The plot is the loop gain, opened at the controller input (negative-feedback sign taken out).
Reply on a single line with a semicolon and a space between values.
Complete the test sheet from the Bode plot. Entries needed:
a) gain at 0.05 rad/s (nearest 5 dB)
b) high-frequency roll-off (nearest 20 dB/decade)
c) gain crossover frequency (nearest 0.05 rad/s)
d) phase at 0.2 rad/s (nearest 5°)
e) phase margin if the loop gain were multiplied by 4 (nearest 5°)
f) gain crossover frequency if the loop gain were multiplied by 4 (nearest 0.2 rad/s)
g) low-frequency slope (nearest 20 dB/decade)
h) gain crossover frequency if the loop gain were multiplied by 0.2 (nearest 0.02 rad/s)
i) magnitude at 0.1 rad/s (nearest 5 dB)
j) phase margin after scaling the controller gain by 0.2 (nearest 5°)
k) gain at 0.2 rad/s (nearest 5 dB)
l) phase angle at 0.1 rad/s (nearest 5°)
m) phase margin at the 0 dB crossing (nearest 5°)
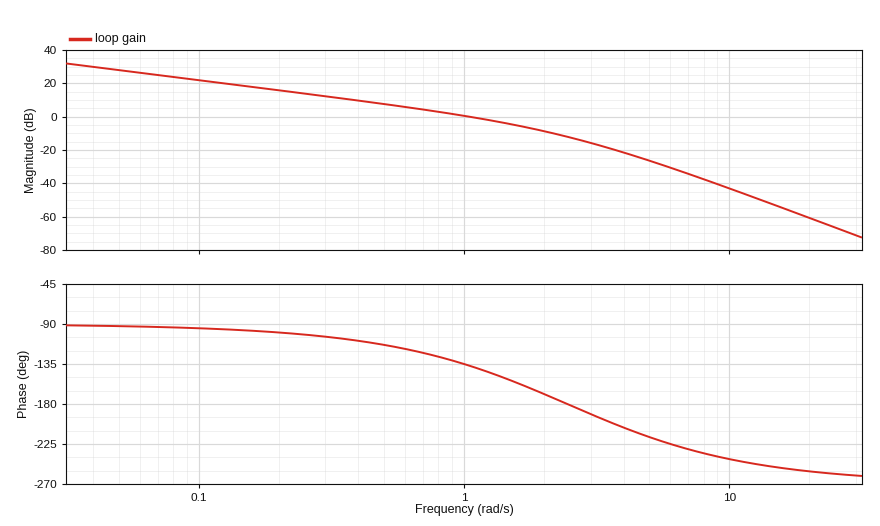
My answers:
30 dB; -60 dB/decade; 1.05 rad/s; -100°; 0°; 2.4 rad/s; -20 dB/decade; 0.24 rad/s; 20 dB; 80°; 15 dB; -95°; 45°
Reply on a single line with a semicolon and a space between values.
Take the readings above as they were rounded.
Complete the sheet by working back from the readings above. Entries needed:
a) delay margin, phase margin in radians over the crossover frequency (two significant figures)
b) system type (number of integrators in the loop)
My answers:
0.75 s; 1
